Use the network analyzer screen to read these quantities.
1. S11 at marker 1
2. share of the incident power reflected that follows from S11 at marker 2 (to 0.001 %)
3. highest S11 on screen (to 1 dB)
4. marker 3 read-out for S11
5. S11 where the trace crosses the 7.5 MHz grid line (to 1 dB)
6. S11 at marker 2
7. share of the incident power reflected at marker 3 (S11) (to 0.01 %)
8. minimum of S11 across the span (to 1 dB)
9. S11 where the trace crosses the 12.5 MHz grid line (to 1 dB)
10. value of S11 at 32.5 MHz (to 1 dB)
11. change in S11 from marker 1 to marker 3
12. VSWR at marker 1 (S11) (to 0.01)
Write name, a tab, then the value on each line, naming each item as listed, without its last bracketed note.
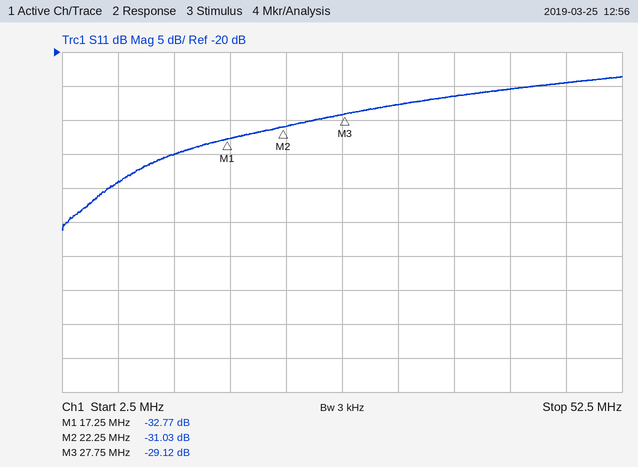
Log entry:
S11 at marker 1	-32.77 dB
share of the incident power reflected that follows from S11 at marker 2	0.079 %
highest S11 on screen	-24 dB
marker 3 read-out for S11	-29.12 dB
S11 where the trace crosses the 7.5 MHz grid line	-39 dB
S11 at marker 2	-31.03 dB
share of the incident power reflected at marker 3 (S11)	0.12 %
minimum of S11 across the span	-46 dB
S11 where the trace crosses the 12.5 MHz grid line	-35 dB
value of S11 at 32.5 MHz	-28 dB
change in S11 from marker 1 to marker 3	3.65 dB
VSWR at marker 1 (S11)	1.05
